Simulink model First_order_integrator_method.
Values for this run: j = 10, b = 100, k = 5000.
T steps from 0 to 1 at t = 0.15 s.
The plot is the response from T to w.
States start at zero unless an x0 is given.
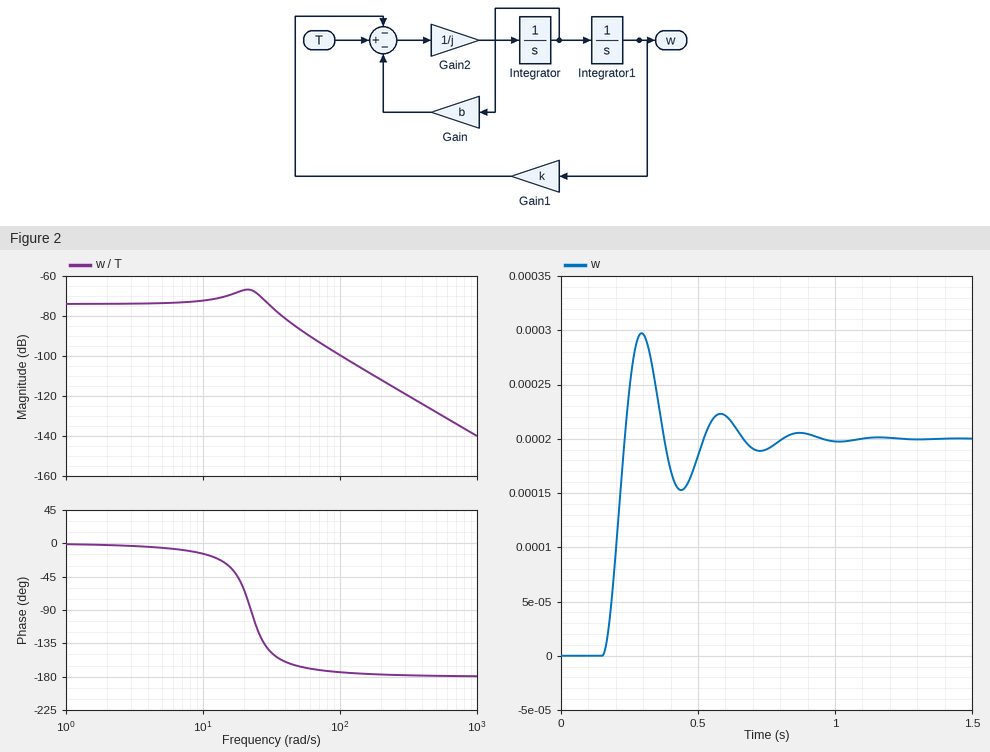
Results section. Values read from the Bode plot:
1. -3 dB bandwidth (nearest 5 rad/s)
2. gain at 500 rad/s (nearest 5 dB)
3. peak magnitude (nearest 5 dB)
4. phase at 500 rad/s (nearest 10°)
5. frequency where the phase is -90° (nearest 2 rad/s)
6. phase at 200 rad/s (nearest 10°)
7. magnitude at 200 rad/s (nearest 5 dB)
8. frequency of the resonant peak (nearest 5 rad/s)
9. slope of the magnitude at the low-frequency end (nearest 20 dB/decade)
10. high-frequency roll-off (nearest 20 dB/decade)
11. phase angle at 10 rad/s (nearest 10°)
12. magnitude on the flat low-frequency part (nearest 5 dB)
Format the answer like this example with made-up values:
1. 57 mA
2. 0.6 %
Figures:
1. 35 rad/s
2. -130 dB
3. -65 dB
4. -180°
5. 22 rad/s
6. -180°
7. -110 dB
8. 20 rad/s
9. 0 dB/decade
10. -40 dB/decade
11. -10°
12. -75 dB
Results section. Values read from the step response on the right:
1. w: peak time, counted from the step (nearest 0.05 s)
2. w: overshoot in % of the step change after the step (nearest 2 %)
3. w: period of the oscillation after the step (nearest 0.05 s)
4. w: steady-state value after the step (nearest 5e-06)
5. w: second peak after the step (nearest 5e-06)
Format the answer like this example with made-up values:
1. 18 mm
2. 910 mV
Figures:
1. 0.15 s
2. 48 %
3. 0.30 s
4. 0.000200
5. 0.000225
